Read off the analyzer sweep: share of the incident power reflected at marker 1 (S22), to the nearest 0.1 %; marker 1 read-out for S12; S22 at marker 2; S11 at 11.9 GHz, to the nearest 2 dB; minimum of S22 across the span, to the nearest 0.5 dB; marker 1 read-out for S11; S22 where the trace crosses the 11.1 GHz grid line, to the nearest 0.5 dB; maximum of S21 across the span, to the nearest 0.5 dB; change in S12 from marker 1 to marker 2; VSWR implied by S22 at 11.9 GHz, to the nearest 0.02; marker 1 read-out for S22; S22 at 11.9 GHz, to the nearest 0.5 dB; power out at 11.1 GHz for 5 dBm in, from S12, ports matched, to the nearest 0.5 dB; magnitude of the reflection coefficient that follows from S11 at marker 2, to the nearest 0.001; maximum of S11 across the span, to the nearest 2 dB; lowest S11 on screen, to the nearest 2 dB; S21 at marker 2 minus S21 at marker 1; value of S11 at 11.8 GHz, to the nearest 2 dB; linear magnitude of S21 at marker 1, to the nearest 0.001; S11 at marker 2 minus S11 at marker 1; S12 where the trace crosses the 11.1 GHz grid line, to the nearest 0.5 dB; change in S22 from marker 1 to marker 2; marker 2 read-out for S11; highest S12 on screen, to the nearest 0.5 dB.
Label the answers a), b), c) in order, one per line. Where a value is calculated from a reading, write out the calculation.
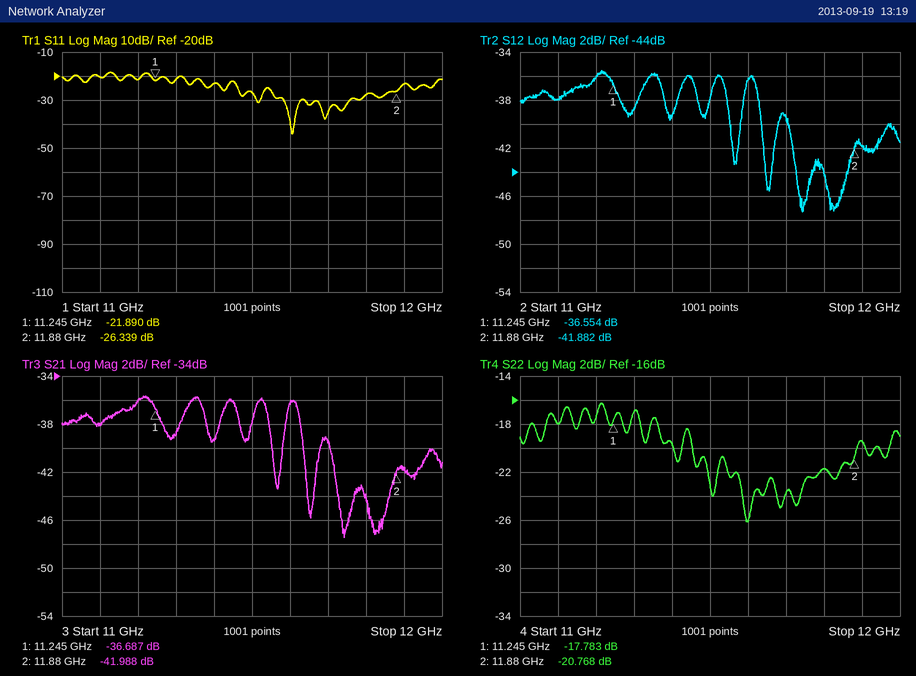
a) 10^(-17.783/10) ≈ 1.7 %
b) -36.554 dB
c) -20.768 dB
d) -24 dB
e) -26.0 dB
f) -21.890 dB
g) -18.0 dB
h) -35.5 dB
i) -41.882 − (-36.554) = -5.328 dB
j) |Γ| = 10^(-19.5/20) = 0.1059; VSWR = (1 + 0.1059)/(1 − 0.1059) ≈ 1.24
k) -17.783 dB
l) -19.5 dB
m) 5 dBm + (-38.0 dB) = -33.0 dBm
n) 10^(-26.339/20) ≈ 0.048
o) -18 dB
p) -44 dB
q) -41.988 − (-36.687) = -5.301 dB
r) -28 dB
s) 10^(-36.687/20) ≈ 0.015
t) -26.339 − (-21.89) = -4.449 dB
u) -38.0 dB
v) -20.768 − (-17.783) = -2.985 dB
w) -26.339 dB
x) -35.5 dB
